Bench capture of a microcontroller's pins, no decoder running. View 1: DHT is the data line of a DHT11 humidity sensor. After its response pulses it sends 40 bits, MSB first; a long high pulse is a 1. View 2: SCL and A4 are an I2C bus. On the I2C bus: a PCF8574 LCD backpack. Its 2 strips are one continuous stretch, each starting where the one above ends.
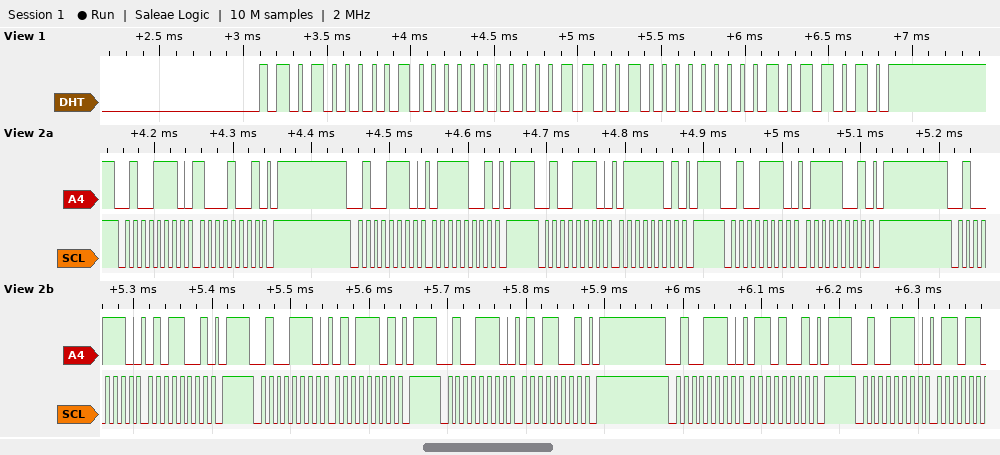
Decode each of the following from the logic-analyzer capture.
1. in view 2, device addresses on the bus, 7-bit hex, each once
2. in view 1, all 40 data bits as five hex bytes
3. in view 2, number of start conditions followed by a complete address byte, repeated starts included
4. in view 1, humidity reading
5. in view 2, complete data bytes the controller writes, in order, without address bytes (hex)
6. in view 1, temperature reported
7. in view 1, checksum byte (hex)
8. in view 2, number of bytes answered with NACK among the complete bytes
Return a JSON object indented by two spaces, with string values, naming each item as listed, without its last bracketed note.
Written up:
{
  "in view 2, device addresses on the bus, 7-bit hex, each once": "0x27",
  "in view 1, all 40 data bits as five hex bytes": "41 00 19 00 5A",
  "in view 2, number of start conditions followed by a complete address byte, repeated starts included": "9",
  "in view 1, humidity reading": "65 %",
  "in view 2, complete data bytes the controller writes, in order, without address bytes": "89 79 7D 79 59 5D 59 69",
  "in view 1, temperature reported": "25.0 °C",
  "in view 1, checksum byte": "0x5A",
  "in view 2, number of bytes answered with NACK among the complete bytes": "0"
}
